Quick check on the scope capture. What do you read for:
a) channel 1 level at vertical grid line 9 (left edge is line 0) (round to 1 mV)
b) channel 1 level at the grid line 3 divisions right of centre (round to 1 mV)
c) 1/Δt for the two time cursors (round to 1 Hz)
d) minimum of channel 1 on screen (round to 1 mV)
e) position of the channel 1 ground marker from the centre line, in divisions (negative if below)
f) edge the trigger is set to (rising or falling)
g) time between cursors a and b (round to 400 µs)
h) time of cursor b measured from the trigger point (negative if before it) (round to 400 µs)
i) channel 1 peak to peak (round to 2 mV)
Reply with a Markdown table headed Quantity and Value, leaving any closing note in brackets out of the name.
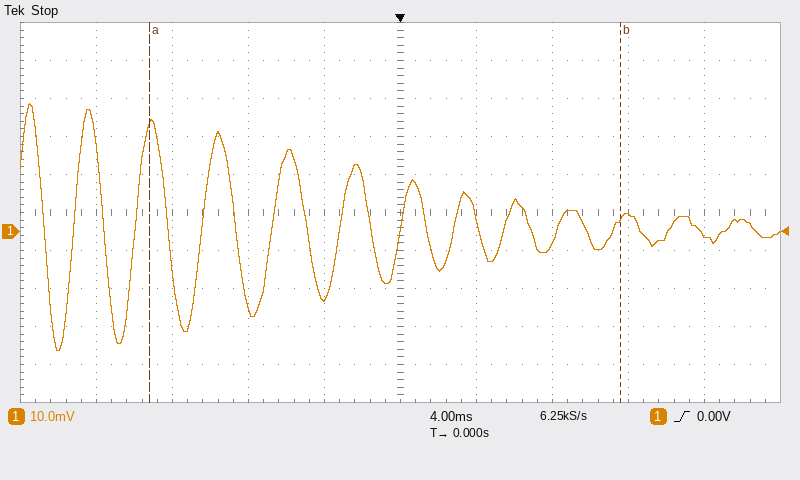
| Quantity | Value |
|---|---|
| channel 1 level at vertical grid line 9 (left edge is line 0) | -1 mV |
| channel 1 level at the grid line 3 divisions right of centre | 4 mV |
| 1/Δt for the two time cursors | 40 Hz |
| minimum of channel 1 on screen | -31 mV |
| position of the channel 1 ground marker from the centre line, in divisions | -0.5 div |
| edge the trigger is set to | rising |
| time between cursors a and b | 24.8 ms |
| time of cursor b measured from the trigger point (negative if before it) | +11.6 ms |
| channel 1 peak to peak | 64 mV |
